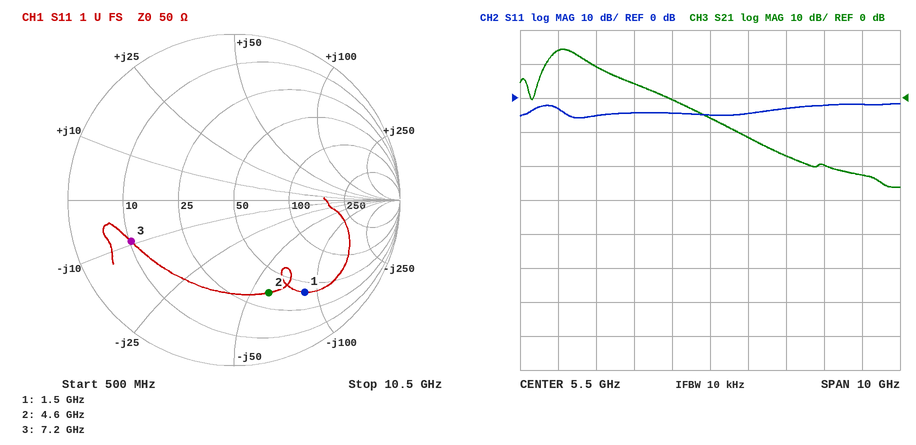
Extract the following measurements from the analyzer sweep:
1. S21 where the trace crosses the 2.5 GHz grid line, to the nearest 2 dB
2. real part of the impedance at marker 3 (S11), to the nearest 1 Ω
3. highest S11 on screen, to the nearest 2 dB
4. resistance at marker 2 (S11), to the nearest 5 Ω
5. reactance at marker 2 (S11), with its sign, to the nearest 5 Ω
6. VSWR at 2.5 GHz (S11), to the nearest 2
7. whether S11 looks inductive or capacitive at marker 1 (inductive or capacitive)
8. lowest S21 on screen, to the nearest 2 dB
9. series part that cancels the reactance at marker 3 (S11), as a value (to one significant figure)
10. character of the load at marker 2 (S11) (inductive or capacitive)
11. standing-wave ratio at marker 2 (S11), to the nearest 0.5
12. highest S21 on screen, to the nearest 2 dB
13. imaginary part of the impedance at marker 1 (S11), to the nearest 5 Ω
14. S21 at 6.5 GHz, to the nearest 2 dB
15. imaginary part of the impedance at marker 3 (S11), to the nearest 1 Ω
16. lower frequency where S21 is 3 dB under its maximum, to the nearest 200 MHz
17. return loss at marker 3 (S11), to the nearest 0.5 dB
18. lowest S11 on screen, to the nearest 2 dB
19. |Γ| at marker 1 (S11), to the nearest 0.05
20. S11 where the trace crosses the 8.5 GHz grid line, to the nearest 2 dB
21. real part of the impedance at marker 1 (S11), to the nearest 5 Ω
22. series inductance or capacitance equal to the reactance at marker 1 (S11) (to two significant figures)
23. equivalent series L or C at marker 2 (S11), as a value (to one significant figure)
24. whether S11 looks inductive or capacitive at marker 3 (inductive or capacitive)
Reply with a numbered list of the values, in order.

1. 10 dB
2. 10 Ω
3. -2 dB
4. 35 Ω
5. -60 Ω
6. 4
7. capacitive
8. -26 dB
9. 200 pH
10. capacitive
11. 4.0
12. 14 dB
13. -85 Ω
14. -12 dB
15. -9 Ω
16. 1.2 GHz
17. 3.5 dB
18. -6 dB
19. 0.70
20. -2 dB
21. 40 Ω
22. 1.2 pF
23. 600 fF
24. capacitive
